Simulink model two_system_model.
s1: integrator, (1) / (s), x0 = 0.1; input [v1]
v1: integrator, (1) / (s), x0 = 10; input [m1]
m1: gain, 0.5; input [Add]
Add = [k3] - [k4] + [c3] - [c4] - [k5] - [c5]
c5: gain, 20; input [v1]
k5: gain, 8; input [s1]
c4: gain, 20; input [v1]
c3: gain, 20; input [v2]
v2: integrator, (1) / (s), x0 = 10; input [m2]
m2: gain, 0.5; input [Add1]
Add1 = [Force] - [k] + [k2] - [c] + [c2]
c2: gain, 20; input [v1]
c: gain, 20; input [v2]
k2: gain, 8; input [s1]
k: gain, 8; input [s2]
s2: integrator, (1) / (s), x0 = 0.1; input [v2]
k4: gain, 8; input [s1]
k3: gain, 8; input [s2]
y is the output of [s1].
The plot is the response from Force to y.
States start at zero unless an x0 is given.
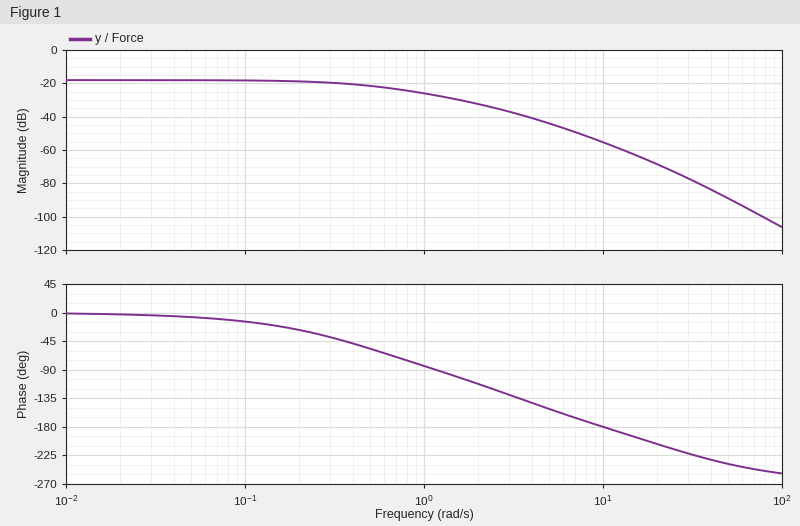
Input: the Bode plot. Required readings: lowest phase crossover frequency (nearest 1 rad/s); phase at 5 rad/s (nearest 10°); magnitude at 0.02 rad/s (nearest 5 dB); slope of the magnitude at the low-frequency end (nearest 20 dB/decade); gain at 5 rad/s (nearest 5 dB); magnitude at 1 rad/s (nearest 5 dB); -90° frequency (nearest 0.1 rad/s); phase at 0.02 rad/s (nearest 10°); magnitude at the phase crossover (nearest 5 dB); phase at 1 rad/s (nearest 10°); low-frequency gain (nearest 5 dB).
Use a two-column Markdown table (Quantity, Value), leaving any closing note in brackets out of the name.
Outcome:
| Quantity | Value |
|---|---|
| lowest phase crossover frequency | 10 rad/s |
| phase at 5 rad/s | -150° |
| magnitude at 0.02 rad/s | -20 dB |
| slope of the magnitude at the low-frequency end | 0 dB/decade |
| gain at 5 rad/s | -45 dB |
| magnitude at 1 rad/s | -25 dB |
| -90° frequency | 1.2 rad/s |
| phase at 0.02 rad/s | 0° |
| magnitude at the phase crossover | -55 dB |
| phase at 1 rad/s | -80° |
| low-frequency gain | -20 dB |
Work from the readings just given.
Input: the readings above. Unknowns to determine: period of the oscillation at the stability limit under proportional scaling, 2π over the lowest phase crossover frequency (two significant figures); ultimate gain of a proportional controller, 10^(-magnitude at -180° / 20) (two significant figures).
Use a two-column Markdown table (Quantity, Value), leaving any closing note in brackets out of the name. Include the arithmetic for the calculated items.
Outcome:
| Quantity | Value |
|---|---|
| period of the oscillation at the stability limit under proportional scaling, 2π over the lowest phase crossover frequency | 2π / 10 = 0.63 s |
| ultimate gain of a proportional controller, 10^(-magnitude at -180° / 20) | 10^(55 / 20) = 560 |
